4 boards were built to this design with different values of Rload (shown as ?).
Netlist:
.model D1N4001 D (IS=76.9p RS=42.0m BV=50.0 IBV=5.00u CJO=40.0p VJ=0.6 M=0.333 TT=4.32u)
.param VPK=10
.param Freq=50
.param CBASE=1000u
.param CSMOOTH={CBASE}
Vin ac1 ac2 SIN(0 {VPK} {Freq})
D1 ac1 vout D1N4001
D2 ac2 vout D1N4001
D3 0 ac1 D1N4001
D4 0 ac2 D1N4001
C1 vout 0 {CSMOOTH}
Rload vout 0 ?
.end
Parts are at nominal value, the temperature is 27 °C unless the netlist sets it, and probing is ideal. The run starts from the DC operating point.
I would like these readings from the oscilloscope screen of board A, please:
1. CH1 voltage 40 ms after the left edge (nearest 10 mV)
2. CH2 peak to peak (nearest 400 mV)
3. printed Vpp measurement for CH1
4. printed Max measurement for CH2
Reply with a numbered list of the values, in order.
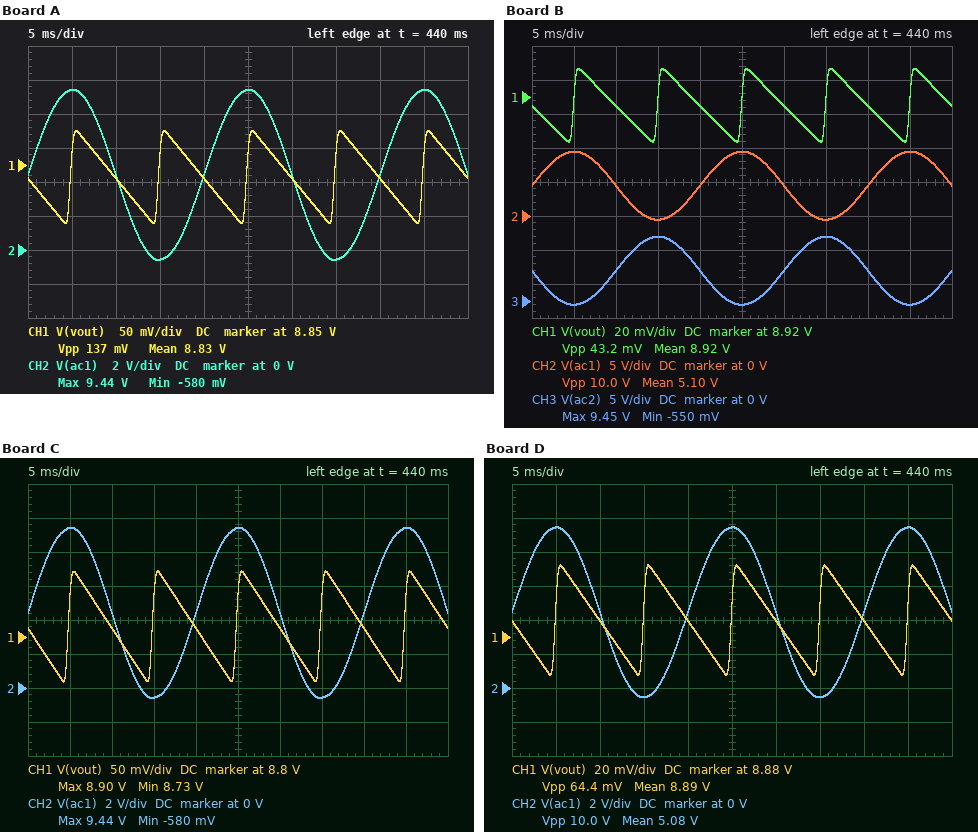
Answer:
1. 8.83 V
2. 10.0 V
3. 137 mV
4. 9.44 V
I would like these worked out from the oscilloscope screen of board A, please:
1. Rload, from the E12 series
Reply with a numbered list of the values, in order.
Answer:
1. 560 Ω
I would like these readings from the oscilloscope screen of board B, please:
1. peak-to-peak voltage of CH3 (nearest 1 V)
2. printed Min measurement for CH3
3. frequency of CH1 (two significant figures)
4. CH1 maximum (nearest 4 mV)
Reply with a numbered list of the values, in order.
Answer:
1. 10 V
2. -550 mV
3. 100 Hz
4. 8.936 V
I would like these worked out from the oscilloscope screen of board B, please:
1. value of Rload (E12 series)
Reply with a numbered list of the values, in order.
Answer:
1. 1.8 kΩ
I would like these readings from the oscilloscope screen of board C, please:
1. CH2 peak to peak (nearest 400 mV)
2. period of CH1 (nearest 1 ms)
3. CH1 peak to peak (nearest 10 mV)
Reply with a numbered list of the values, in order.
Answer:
1. 10.0 V
2. 10 ms
3. 160 mV
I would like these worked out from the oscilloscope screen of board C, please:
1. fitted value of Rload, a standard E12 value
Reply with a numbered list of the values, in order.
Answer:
1. 470 Ω
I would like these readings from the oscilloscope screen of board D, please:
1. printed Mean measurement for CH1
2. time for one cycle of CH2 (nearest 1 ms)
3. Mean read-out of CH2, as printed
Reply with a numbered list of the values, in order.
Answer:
1. 8.89 V
2. 20 ms
3. 5.08 V
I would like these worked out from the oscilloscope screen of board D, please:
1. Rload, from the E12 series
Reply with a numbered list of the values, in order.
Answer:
1. 1.2 kΩ
